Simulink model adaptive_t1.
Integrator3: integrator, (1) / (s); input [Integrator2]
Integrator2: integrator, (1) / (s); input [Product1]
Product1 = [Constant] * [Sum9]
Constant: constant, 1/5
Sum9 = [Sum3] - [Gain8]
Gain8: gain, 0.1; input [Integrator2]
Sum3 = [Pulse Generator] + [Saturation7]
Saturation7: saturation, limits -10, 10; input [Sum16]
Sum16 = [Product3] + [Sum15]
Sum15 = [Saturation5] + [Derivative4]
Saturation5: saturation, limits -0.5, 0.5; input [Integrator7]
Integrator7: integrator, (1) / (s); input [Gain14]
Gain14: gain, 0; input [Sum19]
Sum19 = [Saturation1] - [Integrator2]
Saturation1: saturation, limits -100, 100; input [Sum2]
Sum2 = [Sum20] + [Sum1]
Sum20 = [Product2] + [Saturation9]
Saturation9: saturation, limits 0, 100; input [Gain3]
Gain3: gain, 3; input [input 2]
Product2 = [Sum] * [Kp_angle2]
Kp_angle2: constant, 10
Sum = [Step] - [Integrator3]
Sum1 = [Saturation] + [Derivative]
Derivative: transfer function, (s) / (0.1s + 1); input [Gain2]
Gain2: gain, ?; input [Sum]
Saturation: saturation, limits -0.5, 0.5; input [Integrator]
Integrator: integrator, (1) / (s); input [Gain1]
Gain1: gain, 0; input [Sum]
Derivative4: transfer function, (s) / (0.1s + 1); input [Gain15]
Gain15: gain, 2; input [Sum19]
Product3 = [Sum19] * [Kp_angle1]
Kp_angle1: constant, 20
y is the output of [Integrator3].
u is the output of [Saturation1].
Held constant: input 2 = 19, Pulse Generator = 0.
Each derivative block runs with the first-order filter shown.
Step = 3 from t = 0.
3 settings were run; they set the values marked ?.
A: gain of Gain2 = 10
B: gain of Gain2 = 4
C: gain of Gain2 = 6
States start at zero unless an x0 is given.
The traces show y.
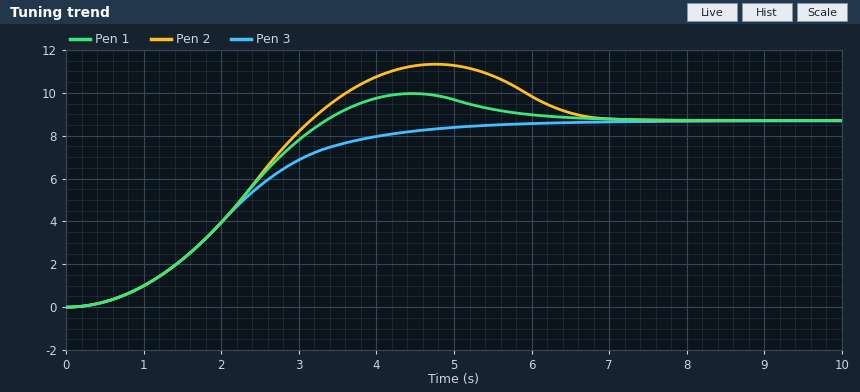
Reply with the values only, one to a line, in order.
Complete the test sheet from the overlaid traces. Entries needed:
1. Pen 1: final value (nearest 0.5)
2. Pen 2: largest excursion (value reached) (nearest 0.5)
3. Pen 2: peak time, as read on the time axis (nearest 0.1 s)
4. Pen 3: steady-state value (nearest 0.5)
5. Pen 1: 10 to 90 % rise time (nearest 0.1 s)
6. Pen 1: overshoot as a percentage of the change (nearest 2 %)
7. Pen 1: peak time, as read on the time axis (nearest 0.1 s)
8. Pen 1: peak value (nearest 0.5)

8.5
11.5
4.8 s
8.5
2.1 s
14 %
4.5 s
10.0
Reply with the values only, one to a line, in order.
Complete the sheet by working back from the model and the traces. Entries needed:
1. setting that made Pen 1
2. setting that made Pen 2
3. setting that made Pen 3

C
B
A
